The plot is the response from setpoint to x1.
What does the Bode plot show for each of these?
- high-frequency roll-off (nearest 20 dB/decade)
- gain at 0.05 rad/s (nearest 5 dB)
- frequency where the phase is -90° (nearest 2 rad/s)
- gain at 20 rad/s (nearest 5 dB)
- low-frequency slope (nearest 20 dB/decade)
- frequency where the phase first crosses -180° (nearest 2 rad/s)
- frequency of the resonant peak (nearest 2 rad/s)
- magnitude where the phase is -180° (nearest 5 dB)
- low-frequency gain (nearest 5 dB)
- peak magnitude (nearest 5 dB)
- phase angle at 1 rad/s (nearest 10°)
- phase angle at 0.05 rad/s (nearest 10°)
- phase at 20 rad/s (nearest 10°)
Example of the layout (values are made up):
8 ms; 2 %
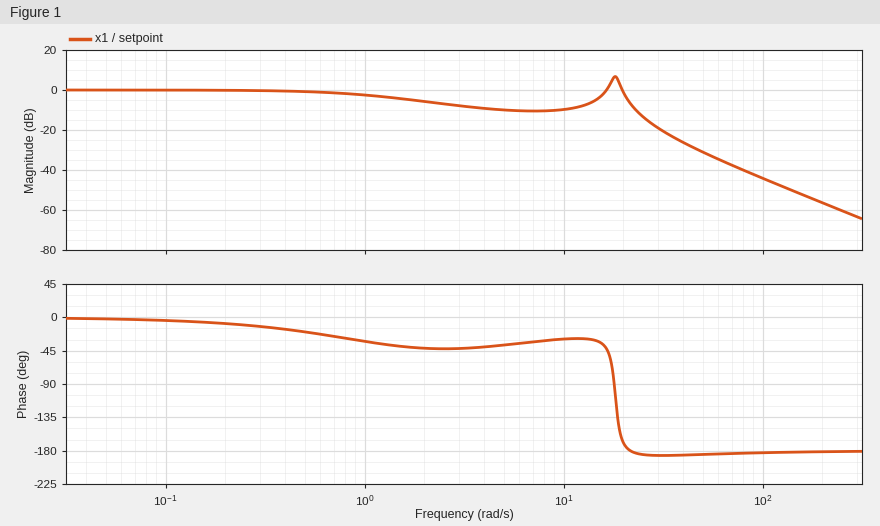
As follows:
-40 dB/decade; 0 dB; 18 rad/s; 0 dB; 0 dB/decade; 22 rad/s; 18 rad/s; -5 dB; 0 dB; 5 dB; -30°; 0°; -170°
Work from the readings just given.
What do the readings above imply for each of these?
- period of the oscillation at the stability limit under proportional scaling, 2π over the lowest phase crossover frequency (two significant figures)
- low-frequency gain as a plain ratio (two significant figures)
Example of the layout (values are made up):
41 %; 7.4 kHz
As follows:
0.29 s; 1.0
